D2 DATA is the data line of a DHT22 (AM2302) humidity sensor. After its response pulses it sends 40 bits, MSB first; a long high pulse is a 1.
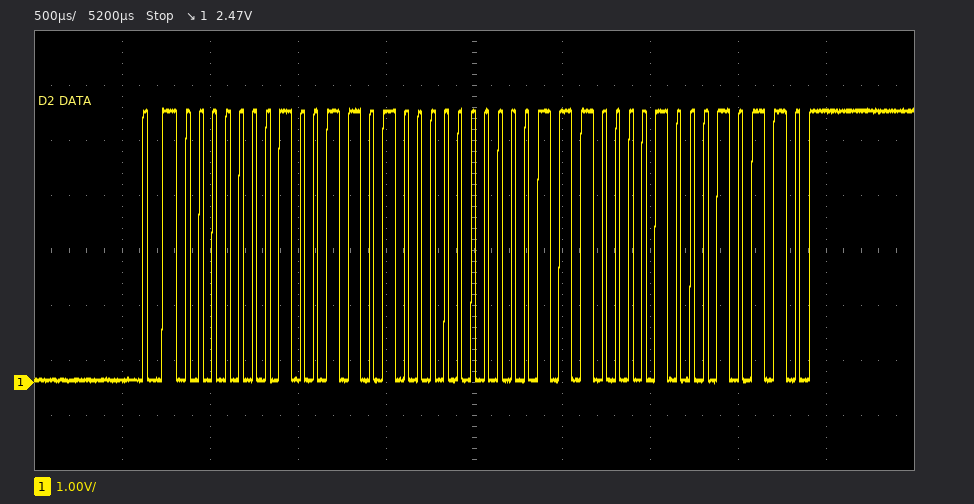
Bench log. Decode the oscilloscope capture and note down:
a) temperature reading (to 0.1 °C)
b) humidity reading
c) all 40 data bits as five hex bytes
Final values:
22.5 °C
30.8 %
01 34 00 E1 16
